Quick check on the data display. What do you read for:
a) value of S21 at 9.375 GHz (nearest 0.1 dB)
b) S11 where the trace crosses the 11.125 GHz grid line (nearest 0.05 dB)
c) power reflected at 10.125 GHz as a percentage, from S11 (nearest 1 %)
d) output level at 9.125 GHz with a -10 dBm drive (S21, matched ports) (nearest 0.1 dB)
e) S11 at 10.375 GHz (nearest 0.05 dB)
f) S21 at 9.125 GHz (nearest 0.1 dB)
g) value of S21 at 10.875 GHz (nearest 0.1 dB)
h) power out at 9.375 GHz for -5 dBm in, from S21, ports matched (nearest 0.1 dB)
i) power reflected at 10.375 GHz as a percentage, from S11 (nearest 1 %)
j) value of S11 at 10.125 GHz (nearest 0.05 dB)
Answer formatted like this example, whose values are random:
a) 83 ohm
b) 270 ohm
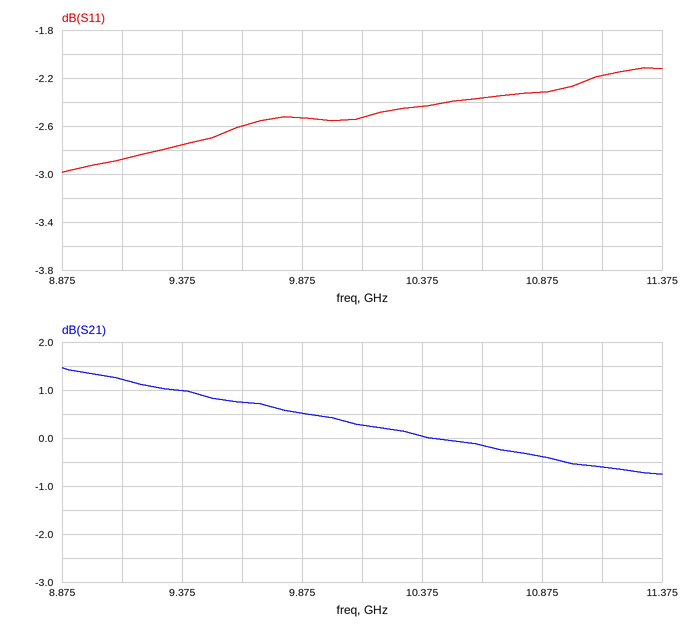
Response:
a) 1.0 dB
b) -2.20 dB
c) 56 %
d) -8.8 dBm
e) -2.45 dB
f) 1.2 dB
g) -0.4 dB
h) -4.0 dBm
i) 57 %
j) -2.55 dB
